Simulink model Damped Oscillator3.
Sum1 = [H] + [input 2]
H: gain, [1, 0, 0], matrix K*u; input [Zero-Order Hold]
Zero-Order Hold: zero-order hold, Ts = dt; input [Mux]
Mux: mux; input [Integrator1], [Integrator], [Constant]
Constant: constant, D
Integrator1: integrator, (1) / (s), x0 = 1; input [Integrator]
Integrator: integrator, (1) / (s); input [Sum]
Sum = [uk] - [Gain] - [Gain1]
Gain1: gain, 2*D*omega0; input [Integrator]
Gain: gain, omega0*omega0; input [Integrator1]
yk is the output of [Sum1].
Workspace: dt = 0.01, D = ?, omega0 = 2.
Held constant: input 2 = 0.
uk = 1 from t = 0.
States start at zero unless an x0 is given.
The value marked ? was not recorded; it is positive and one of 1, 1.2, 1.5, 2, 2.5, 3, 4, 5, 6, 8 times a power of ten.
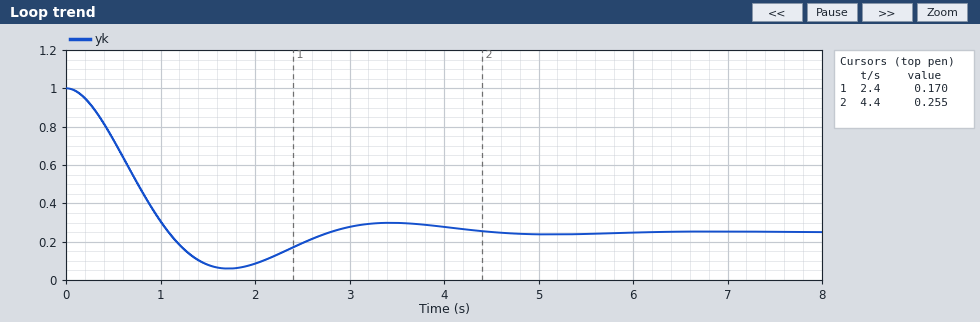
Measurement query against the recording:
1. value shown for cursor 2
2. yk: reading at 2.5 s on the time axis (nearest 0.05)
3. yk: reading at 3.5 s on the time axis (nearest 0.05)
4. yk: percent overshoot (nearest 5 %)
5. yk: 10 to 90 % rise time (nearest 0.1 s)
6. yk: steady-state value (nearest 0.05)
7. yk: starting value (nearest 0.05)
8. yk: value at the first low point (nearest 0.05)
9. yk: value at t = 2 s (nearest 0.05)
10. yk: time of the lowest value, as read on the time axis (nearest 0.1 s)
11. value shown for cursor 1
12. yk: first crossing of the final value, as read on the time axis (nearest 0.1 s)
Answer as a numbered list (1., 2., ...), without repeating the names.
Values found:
1. 0.255
2. 0.20
3. 0.30
4. 25 %
5. 0.7 s
6. 0.25
7. 1.00
8. 0.05
9. 0.10
10. 1.7 s
11. 0.170
12. 1.1 s
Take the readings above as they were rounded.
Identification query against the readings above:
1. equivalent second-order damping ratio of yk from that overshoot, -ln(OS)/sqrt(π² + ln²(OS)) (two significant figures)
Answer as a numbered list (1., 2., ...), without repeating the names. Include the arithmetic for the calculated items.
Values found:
1. ln(0.25) = -1.386; 1.386 / sqrt(9.870 + 1.922) = 0.40
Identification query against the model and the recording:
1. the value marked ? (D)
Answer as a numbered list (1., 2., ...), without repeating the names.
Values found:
1. 0.4
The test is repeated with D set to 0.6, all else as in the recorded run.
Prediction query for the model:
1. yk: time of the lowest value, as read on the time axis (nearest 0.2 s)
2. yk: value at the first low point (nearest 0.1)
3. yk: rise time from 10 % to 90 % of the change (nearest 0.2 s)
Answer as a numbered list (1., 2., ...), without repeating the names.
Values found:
1. 2.0 s
2. 0.2
3. 1.0 s
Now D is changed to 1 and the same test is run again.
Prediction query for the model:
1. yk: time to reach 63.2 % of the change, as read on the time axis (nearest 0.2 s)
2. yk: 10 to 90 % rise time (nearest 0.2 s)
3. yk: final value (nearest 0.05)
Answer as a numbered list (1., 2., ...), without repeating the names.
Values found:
1. 1.0 s
2. 1.6 s
3. 0.25
